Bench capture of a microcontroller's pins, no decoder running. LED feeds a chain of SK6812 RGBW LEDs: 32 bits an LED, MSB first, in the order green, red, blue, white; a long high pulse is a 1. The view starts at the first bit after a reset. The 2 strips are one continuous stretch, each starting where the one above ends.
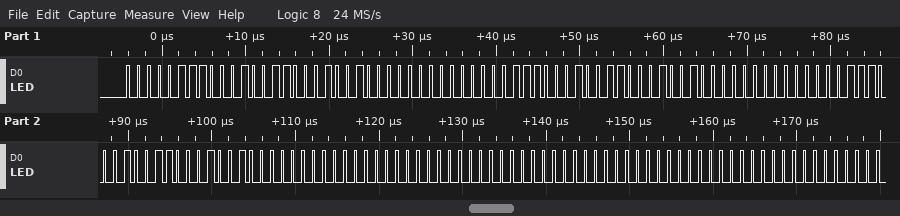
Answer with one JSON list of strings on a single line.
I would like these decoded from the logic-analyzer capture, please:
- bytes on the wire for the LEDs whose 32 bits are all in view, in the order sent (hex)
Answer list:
["07 13 12 00 07 13 12 00 07 13 12 00 00 00 00 00"]
